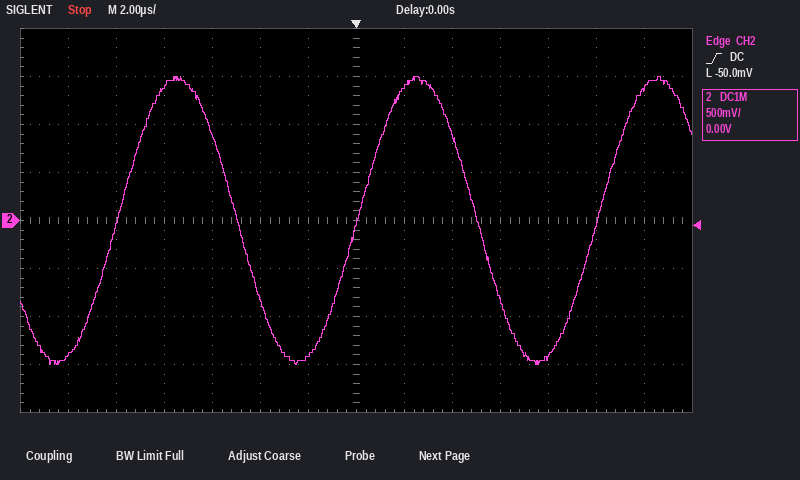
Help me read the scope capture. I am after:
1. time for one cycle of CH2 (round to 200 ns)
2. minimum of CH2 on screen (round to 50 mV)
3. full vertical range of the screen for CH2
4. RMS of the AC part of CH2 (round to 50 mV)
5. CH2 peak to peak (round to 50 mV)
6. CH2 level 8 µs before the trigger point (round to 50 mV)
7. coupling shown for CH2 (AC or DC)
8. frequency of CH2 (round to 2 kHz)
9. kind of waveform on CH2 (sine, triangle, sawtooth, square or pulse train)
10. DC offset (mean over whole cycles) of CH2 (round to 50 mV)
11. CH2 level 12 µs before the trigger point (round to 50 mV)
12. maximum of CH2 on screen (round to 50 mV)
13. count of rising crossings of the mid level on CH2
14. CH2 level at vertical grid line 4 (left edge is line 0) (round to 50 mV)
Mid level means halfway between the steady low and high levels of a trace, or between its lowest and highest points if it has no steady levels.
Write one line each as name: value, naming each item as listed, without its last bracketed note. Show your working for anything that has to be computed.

time for one cycle of CH2: 10.0 µs
minimum of CH2 on screen: -1.50 V
full vertical range of the screen for CH2: 4 V
RMS of the AC part of CH2: 3.00 V / (2√2) ≈ 1.06 V, so 1.05 V to the nearest 50 mV
CH2 peak to peak: 1.50 V − (-1.50 V) = 3.00 V
CH2 level 8 µs before the trigger point: 1.40 V
coupling shown for CH2: DC
frequency of CH2: 1 / 10.0 µs ≈ 100 kHz
kind of waveform on CH2: sine
DC offset (mean over whole cycles) of CH2: (1.50 V + (-1.50 V)) / 2 ≈ 0 mV
CH2 level 12 µs before the trigger point: -1.40 V
maximum of CH2 on screen: 1.50 V
count of rising crossings of the mid level on CH2: 3
CH2 level at vertical grid line 4 (left edge is line 0): 900 mV
